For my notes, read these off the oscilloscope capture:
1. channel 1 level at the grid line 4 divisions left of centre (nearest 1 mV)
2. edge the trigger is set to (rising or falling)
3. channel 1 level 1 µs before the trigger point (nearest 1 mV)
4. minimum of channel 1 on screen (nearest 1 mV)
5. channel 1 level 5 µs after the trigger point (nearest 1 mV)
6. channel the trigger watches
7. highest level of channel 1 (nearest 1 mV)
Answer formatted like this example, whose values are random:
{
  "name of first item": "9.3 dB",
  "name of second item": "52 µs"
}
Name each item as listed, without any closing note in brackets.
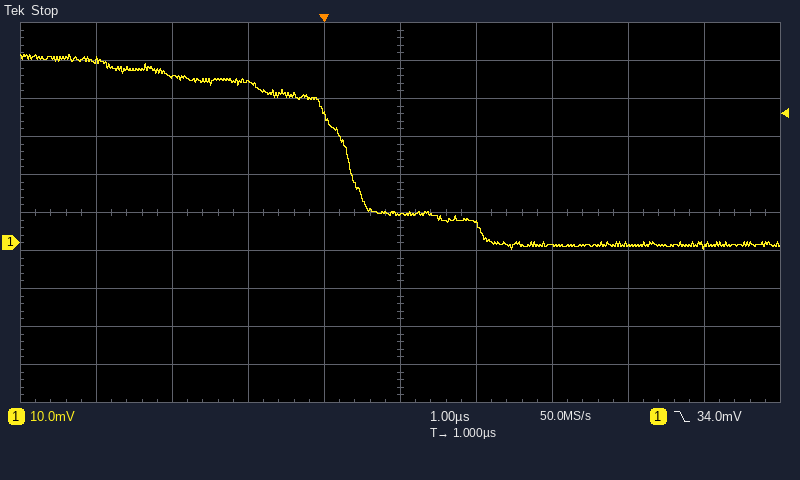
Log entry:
{
  "channel 1 level at the grid line 4 divisions left of centre": "48 mV",
  "edge the trigger is set to": "falling",
  "channel 1 level 1 µs before the trigger point": "42 mV",
  "minimum of channel 1 on screen": "-2 mV",
  "channel 1 level 5 µs after the trigger point": "-1 mV",
  "channel the trigger watches": "channel 1",
  "highest level of channel 1": "50 mV"
}
